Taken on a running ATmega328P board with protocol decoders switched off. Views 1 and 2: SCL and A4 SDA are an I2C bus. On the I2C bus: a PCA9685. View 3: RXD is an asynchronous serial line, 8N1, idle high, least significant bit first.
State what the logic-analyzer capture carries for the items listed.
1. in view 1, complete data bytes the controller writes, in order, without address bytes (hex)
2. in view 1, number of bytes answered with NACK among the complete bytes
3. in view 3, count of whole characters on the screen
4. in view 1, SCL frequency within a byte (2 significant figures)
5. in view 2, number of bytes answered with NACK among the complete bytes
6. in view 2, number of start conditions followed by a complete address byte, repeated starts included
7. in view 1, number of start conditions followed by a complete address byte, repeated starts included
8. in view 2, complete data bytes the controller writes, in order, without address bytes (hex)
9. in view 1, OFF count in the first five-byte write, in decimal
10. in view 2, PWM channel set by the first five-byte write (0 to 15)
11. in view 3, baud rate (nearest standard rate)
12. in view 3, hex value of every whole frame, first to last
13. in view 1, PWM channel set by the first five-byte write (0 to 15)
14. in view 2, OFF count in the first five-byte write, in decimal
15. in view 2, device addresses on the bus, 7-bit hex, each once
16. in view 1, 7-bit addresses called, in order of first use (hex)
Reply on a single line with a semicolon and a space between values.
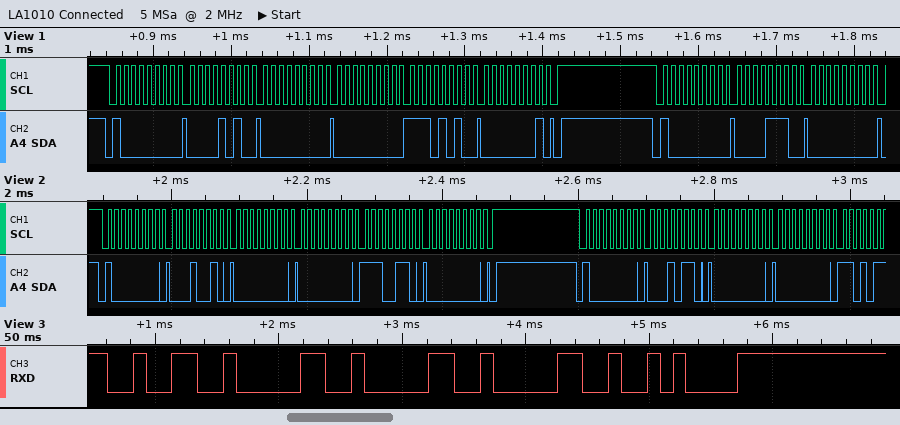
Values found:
0A 00 00 EA 01 0E 00; 0; 5; 100 kHz; 0; 2; 2; 12 00 00 E6 00 16 00 00; 490; 3; 9600 baud; 32 30 30 30 0A; 1; 230; 0x40; 0x40
